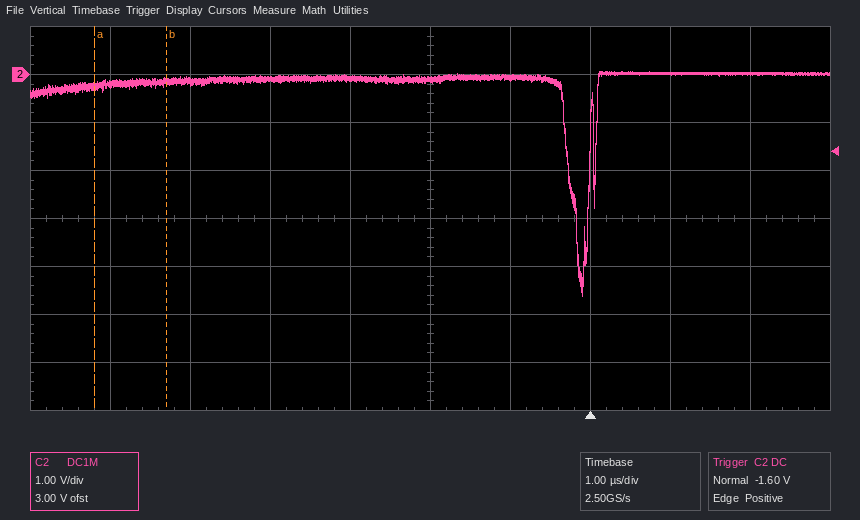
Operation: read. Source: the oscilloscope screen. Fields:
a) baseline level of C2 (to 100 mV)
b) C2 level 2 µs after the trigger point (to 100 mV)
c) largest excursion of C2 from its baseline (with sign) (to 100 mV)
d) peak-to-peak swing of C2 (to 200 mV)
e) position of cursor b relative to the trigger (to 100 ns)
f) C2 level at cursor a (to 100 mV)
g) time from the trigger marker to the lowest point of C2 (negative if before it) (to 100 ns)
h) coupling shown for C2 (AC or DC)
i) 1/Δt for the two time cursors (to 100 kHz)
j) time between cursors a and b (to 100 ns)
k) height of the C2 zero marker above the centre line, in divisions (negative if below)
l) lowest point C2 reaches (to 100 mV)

-100 mV
0.0 V
-4.5 V
4.6 V
-5.3 µs
-200 mV
-100 ns
DC
1.1 MHz
900 ns
+3.0 div
-4.6 V
